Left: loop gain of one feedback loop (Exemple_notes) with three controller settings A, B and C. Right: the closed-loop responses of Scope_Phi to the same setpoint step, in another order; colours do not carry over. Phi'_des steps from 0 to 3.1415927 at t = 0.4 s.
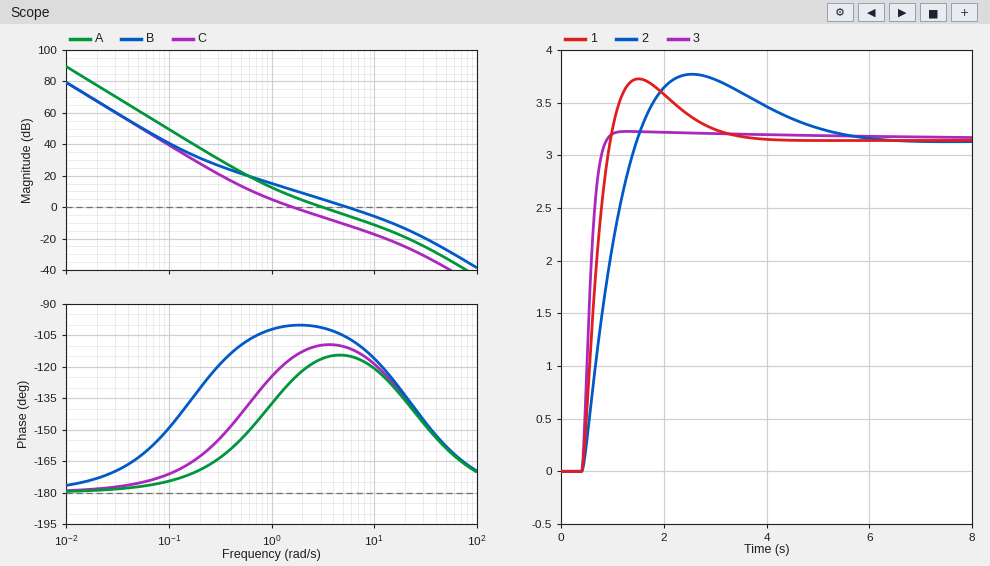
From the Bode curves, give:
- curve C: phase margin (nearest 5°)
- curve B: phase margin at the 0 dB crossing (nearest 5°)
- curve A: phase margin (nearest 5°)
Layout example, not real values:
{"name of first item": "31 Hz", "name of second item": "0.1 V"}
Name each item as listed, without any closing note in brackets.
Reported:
{"curve C: phase margin": "65°", "curve B: phase margin at the 0 dB crossing": "75°", "curve A: phase margin": "65°"}
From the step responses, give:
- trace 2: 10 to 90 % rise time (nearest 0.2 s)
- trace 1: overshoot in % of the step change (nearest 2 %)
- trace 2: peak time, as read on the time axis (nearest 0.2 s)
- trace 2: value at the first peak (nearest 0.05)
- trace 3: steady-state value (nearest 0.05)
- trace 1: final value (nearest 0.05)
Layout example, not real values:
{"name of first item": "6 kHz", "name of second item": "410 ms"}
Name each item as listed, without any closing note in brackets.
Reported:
{"trace 2: 10 to 90 % rise time": "0.8 s", "trace 1: overshoot in % of the step change": "18 %", "trace 2: peak time, as read on the time axis": "2.6 s", "trace 2: value at the first peak": "3.75", "trace 3: steady-state value": "3.15", "trace 1: final value": "3.15"}
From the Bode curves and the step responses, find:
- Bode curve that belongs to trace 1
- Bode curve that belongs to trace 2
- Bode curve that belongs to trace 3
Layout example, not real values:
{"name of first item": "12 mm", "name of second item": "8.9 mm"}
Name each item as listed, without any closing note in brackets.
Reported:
{"Bode curve that belongs to trace 1": "A", "Bode curve that belongs to trace 2": "C", "Bode curve that belongs to trace 3": "B"}
